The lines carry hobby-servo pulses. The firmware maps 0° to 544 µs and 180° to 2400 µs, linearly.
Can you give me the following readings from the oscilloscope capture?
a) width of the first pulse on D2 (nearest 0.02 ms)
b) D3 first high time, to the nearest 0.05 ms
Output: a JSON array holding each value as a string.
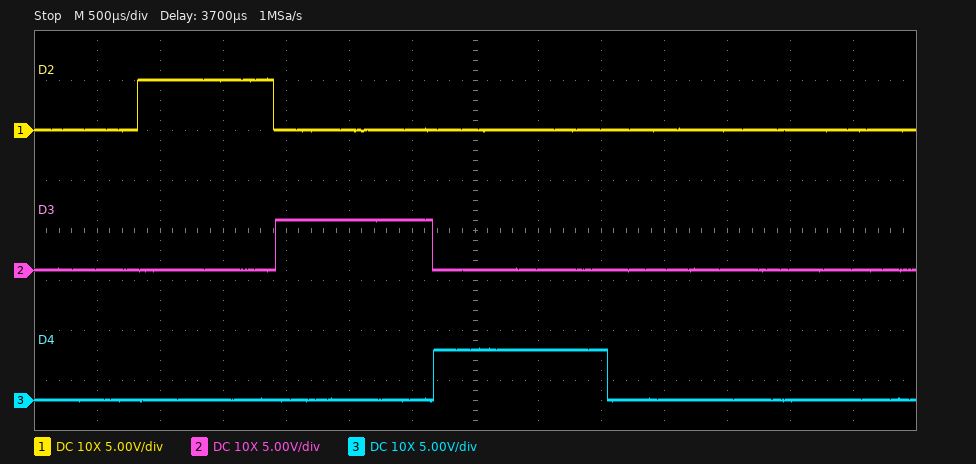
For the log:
["1.08 ms", "1.25 ms"]
